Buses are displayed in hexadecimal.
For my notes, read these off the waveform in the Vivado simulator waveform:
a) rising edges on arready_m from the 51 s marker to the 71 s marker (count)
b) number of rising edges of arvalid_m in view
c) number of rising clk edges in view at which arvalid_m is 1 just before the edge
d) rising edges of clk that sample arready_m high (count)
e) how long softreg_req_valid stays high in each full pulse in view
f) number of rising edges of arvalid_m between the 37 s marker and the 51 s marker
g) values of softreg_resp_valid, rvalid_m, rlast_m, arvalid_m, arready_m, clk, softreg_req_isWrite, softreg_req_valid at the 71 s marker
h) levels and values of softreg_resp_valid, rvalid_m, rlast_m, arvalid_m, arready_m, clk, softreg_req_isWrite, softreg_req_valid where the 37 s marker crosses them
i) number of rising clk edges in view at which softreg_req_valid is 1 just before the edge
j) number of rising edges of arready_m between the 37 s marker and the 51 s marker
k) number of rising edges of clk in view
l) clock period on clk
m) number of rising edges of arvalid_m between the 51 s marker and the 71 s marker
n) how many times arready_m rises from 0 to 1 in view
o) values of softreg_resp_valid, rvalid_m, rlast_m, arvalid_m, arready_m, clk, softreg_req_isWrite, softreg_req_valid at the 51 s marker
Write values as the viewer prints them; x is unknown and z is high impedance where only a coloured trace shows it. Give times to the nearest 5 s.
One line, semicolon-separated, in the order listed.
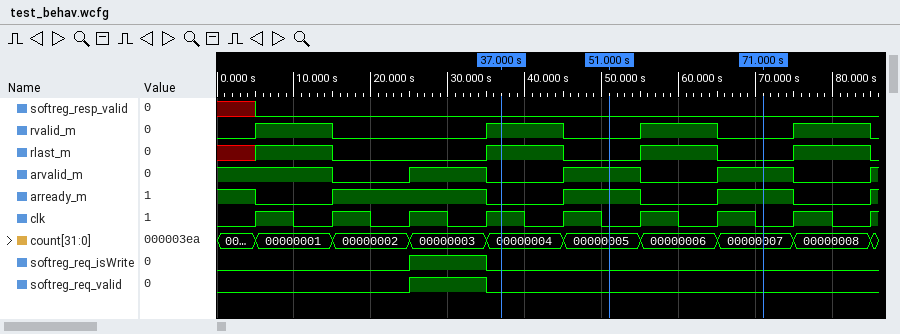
1; 4; 5; 5; 10 s; 1; softreg_resp_valid=0, rvalid_m=0, rlast_m=0, arvalid_m=1, arready_m=1, clk=0, softreg_req_isWrite=0, softreg_req_valid=0; softreg_resp_valid=0, rvalid_m=1, rlast_m=1, arvalid_m=0, arready_m=0, clk=1, softreg_req_isWrite=0, softreg_req_valid=0; 1; 1; 9; 10 s; 1; 4; softreg_resp_valid=0, rvalid_m=0, rlast_m=0, arvalid_m=1, arready_m=1, clk=0, softreg_req_isWrite=0, softreg_req_valid=0
